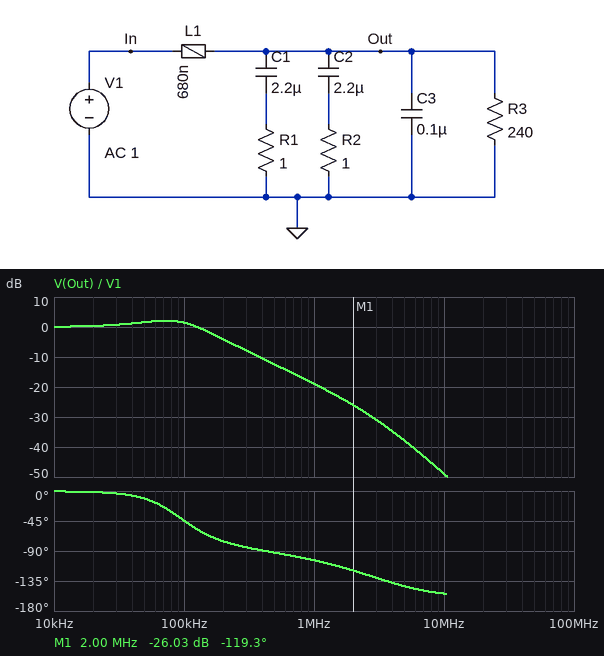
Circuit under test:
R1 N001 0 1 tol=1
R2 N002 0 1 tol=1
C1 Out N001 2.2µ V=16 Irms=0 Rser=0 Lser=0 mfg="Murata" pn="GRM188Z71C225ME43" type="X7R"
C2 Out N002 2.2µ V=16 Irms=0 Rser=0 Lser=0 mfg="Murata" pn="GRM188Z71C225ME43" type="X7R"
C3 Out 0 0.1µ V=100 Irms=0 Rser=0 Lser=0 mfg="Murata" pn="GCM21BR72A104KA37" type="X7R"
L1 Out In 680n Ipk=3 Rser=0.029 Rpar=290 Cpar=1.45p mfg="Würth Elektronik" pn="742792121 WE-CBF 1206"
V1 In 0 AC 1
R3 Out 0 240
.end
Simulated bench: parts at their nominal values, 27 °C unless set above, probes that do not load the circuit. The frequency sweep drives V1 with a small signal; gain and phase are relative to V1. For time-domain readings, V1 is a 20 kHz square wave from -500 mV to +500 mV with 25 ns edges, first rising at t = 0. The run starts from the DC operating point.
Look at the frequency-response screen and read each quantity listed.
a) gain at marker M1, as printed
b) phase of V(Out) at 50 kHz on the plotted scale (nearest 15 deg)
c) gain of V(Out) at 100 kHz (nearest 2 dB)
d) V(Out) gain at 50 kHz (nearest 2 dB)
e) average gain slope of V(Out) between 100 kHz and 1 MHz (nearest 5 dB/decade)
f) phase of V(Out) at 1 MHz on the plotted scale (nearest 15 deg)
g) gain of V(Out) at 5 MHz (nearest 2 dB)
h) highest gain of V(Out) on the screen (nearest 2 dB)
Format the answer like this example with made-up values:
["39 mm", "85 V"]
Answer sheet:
["-26.03 dB", "-15 deg", "2 dB", "2 dB", "-20 dB/decade", "-105 deg", "-38 dB", "2 dB"]
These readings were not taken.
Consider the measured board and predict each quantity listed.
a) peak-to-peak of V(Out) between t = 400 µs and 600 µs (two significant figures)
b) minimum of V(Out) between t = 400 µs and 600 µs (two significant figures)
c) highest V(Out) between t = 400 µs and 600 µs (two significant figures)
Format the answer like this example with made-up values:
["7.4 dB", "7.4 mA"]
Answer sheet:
["1.4 V", "-710 mV", "710 mV"]
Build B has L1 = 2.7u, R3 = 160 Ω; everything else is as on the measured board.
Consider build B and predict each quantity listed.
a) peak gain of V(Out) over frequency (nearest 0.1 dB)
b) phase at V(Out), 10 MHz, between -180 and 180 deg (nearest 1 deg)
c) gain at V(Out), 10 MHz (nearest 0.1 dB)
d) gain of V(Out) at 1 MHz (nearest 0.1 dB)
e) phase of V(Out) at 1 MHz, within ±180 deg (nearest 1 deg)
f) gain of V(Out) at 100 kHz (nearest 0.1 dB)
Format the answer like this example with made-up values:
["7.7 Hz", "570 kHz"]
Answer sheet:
["5.3 dB", "-132 deg", "-59.8 dB", "-31.1 dB", "-106 deg", "-7.5 dB"]
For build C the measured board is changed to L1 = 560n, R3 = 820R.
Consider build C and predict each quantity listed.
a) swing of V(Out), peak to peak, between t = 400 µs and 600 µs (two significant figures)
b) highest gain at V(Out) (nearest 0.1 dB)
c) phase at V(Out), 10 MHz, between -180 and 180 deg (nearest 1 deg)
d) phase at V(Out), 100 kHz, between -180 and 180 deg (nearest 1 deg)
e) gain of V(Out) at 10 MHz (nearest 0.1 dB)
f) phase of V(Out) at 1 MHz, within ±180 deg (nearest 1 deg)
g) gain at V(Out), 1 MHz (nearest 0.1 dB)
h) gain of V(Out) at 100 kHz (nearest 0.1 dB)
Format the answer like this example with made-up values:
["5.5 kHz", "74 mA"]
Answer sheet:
["1.4 V", "1.8 dB", "-155 deg", "-36 deg", "-47.3 dB", "-103 deg", "-17.2 dB", "1.5 dB"]
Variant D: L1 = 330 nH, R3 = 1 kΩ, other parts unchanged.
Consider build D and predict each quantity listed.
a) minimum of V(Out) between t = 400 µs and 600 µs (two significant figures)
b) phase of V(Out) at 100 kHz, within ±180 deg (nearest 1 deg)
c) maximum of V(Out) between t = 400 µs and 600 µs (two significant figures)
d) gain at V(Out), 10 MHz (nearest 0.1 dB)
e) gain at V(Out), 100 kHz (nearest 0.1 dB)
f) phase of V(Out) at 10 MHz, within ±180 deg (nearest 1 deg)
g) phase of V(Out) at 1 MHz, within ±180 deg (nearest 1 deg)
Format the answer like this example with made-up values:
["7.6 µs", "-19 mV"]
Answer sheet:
["-620 mV", "-20 deg", "620 mV", "-42.7 dB", "1.1 dB", "-158 deg", "-97 deg"]
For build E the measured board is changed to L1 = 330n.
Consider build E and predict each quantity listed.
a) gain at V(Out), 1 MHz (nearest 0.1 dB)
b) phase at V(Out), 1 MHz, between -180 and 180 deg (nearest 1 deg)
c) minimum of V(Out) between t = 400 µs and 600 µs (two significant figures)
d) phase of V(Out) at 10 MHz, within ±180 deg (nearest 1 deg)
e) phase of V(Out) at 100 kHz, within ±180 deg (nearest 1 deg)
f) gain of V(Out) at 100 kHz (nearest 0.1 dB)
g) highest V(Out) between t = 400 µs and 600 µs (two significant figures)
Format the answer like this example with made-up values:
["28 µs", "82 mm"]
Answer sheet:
["-12.5 dB", "-97 deg", "-620 mV", "-158 deg", "-20 deg", "1.1 dB", "620 mV"]
